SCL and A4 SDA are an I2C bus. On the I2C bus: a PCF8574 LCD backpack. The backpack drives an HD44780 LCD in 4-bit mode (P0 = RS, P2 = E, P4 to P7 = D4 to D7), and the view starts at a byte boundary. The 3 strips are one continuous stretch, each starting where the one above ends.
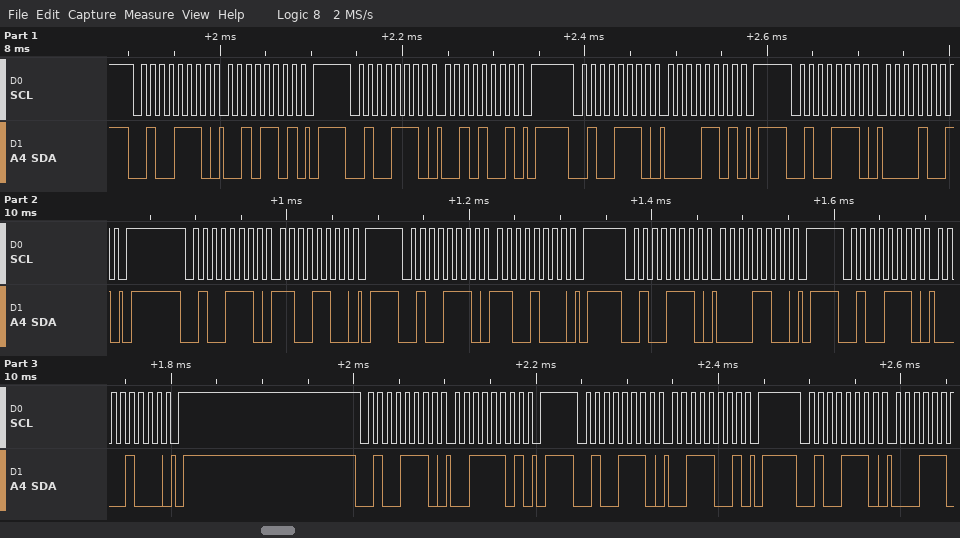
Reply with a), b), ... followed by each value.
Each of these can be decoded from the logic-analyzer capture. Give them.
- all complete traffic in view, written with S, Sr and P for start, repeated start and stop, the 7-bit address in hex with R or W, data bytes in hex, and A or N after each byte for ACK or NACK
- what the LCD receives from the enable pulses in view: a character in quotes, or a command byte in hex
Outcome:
a) S 27W A 2D A P S 27W A 29 A P S 27W A 0D A P S 27W A 09 A P S 27W A CC A P S 27W A C8 A P S 27W A 0C A P S 27W A 08 A P S 27W A 3D A P S 27W A 39 A P S 27W A
b) ' ' 0xC0
